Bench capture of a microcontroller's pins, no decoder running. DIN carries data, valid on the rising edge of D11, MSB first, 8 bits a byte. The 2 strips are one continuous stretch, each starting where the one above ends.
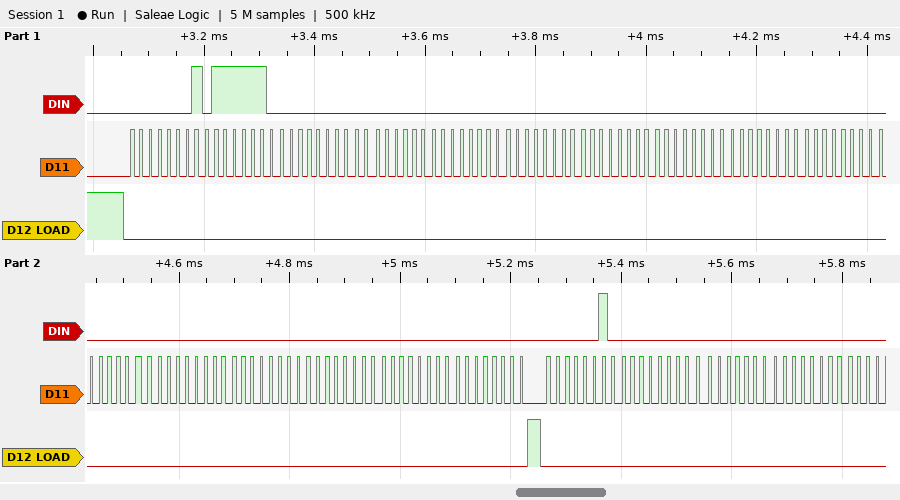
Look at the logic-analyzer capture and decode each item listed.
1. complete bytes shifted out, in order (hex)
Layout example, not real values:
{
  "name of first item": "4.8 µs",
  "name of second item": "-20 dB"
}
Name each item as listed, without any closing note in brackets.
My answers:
{
  "complete bytes shifted out, in order": "0x01 0x7E 0x00 0x00 0x00 0x00 0x00 0x00 0x00 0x00 0x00 0x00 0x00 0x00 0x00 0x00 0x02 0x00 0x00 0x00"
}
